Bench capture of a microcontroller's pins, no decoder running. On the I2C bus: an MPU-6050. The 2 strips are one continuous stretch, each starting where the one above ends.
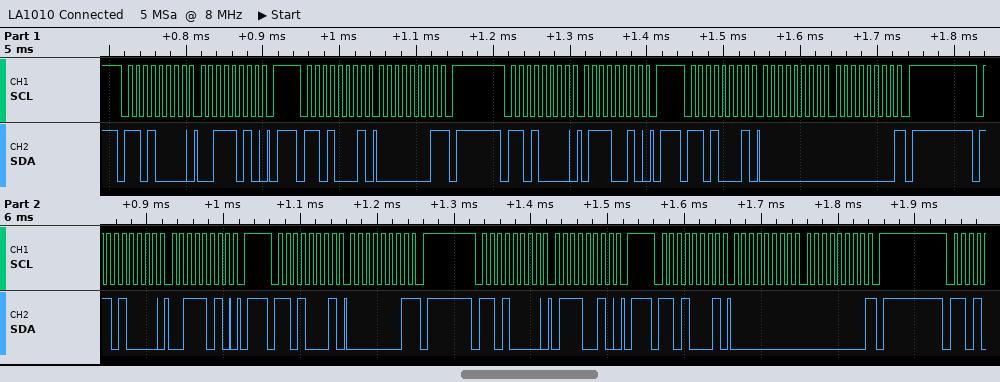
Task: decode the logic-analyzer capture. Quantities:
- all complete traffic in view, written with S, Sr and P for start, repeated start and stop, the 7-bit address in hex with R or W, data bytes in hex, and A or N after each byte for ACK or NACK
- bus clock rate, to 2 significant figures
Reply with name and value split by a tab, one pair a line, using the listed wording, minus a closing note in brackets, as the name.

all complete traffic in view, written with S, Sr and P for start, repeated start and stop, the 7-bit address in hex with R or W, data bytes in hex, and A or N after each byte for ACK or NACK	S 68W A 3A A P S 68R A 01 N P S 68W A 72 A P S 68R A 00 A 00 N P S 68W A 3A A P S 68R A 01 N P S 68W A 72 A P S 68R A 00 A 00 N P
bus clock rate, to 2 significant figures	100 kHz
